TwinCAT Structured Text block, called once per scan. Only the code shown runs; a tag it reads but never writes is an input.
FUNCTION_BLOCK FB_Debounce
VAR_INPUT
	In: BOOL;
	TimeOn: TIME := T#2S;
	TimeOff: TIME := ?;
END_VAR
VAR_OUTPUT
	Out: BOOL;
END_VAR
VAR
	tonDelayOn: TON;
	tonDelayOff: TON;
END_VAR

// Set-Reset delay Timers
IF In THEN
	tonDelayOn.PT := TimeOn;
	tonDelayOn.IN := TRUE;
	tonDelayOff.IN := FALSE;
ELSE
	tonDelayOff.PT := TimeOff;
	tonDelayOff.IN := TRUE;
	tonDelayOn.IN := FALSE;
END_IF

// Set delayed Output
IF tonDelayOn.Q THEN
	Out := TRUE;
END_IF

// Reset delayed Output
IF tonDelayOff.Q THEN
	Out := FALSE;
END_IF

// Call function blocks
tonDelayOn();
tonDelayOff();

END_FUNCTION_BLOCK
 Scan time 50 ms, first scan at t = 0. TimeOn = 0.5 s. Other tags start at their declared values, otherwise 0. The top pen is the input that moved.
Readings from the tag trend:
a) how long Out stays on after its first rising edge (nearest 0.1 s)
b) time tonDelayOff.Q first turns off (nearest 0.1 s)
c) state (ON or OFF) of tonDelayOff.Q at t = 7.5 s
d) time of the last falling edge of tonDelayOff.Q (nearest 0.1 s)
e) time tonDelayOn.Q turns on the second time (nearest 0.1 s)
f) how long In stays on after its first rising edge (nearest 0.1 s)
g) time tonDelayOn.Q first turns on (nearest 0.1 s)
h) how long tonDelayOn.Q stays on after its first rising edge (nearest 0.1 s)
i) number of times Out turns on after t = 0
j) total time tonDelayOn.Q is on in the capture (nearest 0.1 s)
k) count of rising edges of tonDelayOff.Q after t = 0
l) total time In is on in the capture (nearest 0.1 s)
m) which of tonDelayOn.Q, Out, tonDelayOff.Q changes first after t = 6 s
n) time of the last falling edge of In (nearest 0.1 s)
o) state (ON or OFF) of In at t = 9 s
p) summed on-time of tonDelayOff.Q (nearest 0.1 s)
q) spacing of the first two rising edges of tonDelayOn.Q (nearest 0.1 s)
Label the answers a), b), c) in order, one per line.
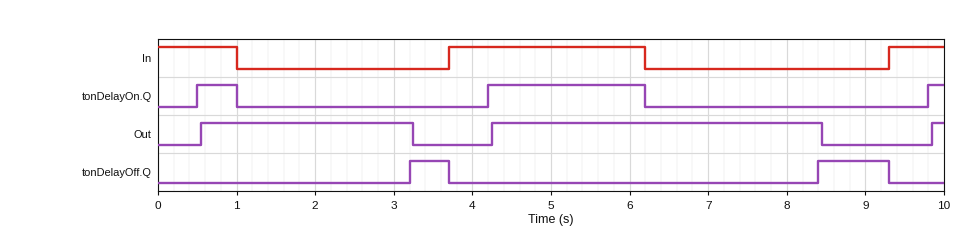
a) 2.7 s
b) 3.7 s
c) OFF
d) 9.3 s
e) 4.2 s
f) 2.5 s
g) 0.5 s
h) 0.5 s
i) 3
j) 2.7 s
k) 2
l) 4.2 s
m) tonDelayOn.Q
n) 6.2 s
o) OFF
p) 1.4 s
q) 3.7 s
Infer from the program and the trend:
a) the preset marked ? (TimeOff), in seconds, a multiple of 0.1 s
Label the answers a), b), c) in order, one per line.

a) 2.2 s
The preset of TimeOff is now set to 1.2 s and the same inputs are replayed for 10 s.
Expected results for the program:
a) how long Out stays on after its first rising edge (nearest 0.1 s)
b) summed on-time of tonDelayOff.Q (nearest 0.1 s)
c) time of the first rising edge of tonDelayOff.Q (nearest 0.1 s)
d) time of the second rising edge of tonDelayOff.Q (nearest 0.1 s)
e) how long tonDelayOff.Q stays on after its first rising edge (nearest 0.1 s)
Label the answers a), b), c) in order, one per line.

a) 1.7 s
b) 3.4 s
c) 2.2 s
d) 7.4 s
e) 1.5 s
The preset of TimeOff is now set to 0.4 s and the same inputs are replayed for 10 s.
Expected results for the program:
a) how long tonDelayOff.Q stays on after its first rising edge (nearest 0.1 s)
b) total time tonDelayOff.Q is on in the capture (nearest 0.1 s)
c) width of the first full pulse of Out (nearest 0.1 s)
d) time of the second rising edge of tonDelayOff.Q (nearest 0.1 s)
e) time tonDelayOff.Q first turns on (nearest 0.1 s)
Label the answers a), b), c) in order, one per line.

a) 2.3 s
b) 5.0 s
c) 0.9 s
d) 6.6 s
e) 1.4 s
